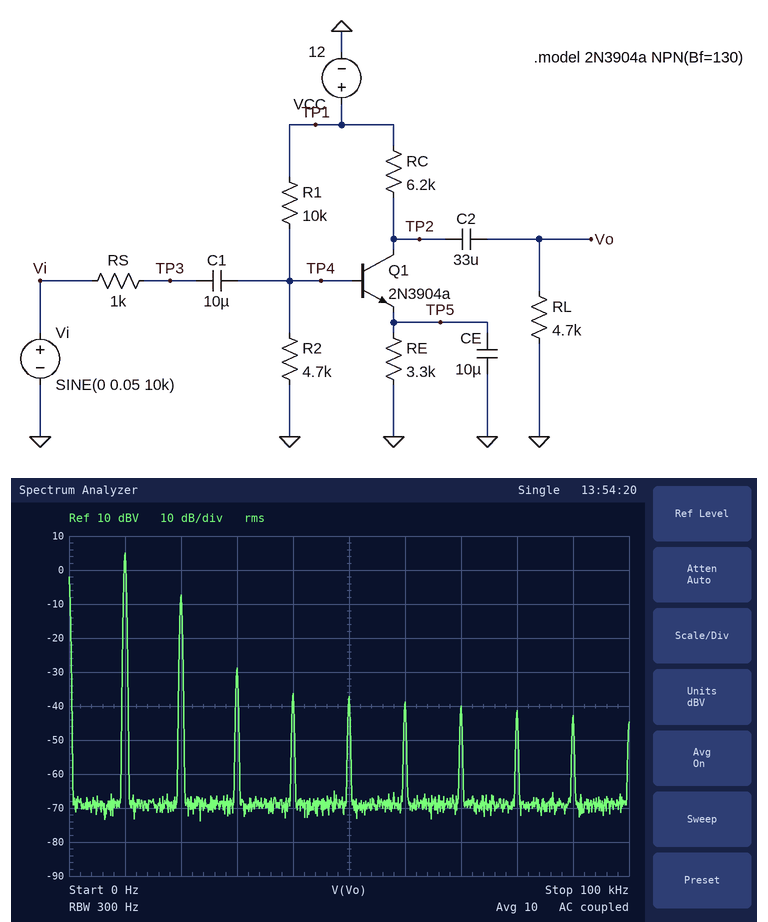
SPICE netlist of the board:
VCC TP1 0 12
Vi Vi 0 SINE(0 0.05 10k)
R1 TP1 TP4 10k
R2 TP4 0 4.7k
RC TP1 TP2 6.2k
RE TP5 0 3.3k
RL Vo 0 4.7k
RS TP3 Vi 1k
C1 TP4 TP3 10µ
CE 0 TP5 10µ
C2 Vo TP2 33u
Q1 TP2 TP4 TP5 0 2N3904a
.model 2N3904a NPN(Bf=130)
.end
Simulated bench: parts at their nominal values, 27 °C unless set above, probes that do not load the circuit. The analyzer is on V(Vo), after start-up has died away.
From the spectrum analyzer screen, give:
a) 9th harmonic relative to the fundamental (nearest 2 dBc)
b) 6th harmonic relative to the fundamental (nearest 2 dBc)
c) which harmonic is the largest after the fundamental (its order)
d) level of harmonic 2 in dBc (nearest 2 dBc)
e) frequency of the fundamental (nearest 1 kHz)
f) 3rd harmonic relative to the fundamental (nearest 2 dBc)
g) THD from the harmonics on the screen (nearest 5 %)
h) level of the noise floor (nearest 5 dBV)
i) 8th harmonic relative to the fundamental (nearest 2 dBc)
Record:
-48 dBc
-44 dBc
2
-12 dBc
10 kHz
-34 dBc
25 %
-70 dBV
-46 dBc
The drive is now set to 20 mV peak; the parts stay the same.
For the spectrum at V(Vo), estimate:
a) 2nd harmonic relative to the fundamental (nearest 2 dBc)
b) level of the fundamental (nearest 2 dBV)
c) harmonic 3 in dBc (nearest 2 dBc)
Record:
-20 dBc
-2 dBV
-48 dBc
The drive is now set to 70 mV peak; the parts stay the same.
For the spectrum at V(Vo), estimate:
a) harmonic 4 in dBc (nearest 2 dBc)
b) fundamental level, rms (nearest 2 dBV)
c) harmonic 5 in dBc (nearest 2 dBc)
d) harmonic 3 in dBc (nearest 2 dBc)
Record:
-22 dBc
6 dBV
-26 dBc
-26 dBc
